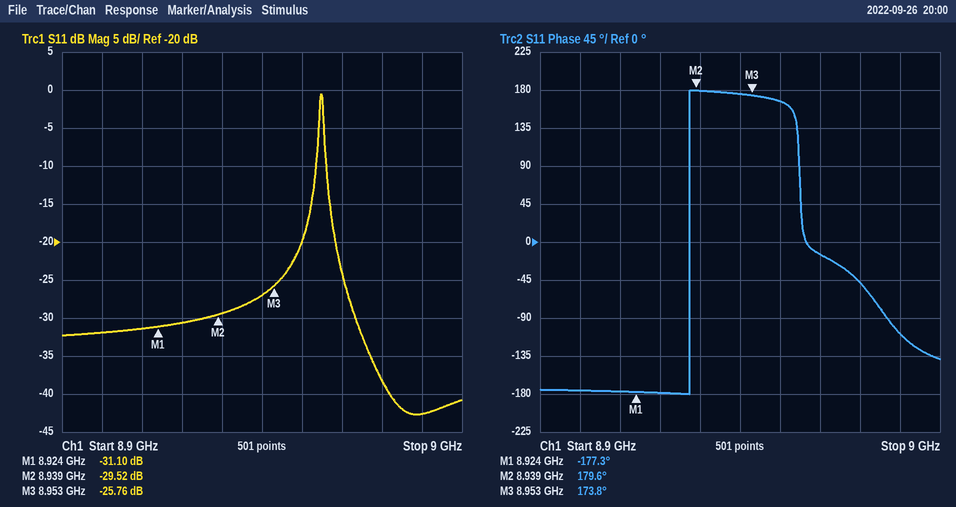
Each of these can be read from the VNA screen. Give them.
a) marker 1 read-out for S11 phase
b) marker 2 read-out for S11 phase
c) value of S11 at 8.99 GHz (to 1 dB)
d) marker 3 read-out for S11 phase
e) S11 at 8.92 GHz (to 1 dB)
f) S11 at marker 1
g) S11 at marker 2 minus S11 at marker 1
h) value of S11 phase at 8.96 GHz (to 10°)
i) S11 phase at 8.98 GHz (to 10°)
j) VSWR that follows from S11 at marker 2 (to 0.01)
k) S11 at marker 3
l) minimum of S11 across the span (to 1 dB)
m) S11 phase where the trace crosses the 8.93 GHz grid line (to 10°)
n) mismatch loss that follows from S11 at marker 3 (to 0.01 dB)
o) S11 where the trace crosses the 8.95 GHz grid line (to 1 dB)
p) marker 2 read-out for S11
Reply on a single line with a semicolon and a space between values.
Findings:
-177.3°; 179.6°; -43 dB; 173.8°; -31 dB; -31.10 dB; 1.58 dB; 170°; -50°; 1.07; -25.76 dB; -43 dB; -180°; 0.01 dB; -27 dB; -29.52 dB
